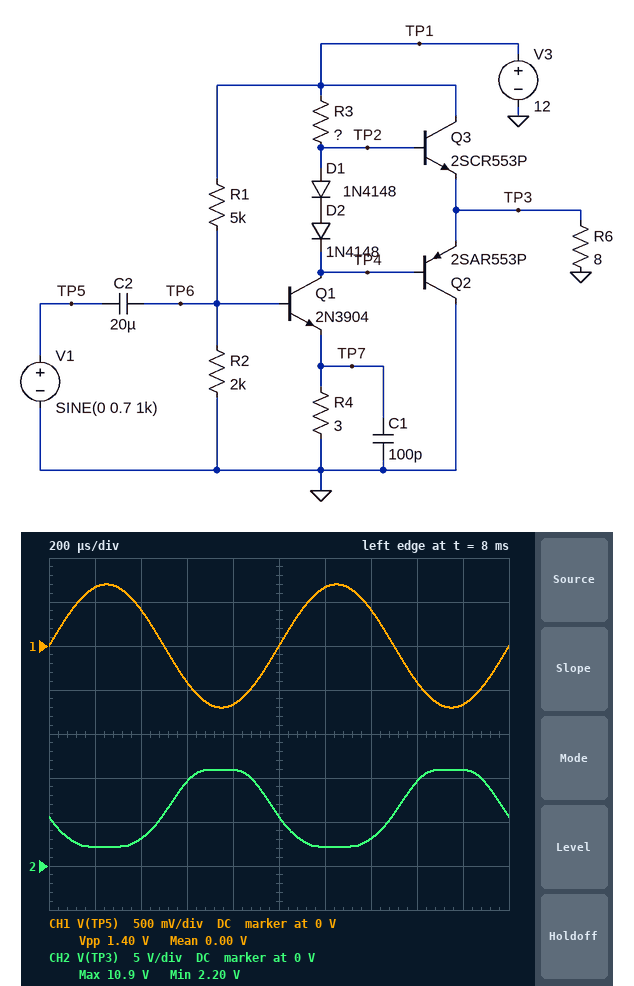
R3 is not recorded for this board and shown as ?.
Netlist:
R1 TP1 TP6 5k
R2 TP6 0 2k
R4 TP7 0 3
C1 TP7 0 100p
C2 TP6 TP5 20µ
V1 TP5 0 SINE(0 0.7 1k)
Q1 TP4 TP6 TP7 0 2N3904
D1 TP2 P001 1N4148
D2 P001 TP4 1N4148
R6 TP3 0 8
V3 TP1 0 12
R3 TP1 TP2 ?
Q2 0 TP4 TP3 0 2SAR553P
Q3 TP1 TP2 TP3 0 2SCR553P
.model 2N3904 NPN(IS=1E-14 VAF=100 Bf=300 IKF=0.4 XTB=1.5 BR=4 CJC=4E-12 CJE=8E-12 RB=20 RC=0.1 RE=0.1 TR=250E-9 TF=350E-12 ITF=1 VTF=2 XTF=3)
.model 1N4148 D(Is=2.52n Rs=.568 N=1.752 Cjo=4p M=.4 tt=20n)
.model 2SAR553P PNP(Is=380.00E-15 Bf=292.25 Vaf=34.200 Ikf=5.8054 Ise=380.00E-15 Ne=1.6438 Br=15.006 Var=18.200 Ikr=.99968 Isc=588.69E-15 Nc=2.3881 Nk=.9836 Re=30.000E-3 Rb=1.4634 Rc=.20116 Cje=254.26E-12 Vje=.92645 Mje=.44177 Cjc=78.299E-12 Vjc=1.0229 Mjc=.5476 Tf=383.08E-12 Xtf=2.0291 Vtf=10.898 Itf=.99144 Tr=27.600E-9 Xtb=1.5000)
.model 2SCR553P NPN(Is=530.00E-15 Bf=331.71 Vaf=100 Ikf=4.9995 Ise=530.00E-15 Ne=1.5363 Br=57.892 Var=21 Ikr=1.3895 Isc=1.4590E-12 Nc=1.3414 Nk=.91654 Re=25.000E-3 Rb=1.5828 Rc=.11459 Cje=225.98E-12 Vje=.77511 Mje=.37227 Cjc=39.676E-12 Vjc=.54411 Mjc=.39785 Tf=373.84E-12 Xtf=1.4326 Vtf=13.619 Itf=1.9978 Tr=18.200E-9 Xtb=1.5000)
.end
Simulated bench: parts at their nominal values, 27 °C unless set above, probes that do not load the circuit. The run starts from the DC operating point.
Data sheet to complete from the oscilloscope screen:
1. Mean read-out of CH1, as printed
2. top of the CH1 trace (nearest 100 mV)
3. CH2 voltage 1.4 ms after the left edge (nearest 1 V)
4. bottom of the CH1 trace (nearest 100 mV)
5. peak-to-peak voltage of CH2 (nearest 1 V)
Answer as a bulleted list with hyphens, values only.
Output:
- 0.00 V
- 700 mV
- 3 V
- -700 mV
- 9 V
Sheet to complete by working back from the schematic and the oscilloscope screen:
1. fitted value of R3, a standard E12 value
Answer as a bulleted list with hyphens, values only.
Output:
- 27 Ω
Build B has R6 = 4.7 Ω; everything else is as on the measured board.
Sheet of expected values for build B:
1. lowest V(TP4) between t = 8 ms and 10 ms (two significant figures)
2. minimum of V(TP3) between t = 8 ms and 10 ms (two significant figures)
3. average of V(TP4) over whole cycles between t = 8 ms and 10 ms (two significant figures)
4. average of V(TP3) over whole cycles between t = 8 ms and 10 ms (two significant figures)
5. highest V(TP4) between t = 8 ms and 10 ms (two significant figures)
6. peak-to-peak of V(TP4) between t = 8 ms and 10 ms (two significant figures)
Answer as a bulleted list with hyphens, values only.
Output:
- 1.1 V
- 2.1 V
- 5.4 V
- 6.1 V
- 10 V
- 9.2 V
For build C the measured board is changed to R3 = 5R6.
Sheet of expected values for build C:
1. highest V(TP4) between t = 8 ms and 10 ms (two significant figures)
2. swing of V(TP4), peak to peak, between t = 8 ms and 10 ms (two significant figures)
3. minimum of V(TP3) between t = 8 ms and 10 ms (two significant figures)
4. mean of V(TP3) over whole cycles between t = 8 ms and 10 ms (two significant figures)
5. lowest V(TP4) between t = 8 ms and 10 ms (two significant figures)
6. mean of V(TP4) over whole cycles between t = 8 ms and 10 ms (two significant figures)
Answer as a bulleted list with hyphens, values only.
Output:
- 10 V
- 3.8 V
- 7.3 V
- 9.1 V
- 6.4 V
- 8.3 V
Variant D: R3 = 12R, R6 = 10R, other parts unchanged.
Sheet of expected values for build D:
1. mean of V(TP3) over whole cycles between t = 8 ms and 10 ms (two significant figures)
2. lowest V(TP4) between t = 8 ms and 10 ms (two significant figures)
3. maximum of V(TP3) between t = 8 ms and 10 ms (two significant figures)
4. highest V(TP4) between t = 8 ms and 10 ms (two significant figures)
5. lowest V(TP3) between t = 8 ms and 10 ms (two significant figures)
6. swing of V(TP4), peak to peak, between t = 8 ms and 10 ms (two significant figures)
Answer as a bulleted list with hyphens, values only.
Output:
- 7.6 V
- 3.9 V
- 11 V
- 10 V
- 4.9 V
- 6.1 V
